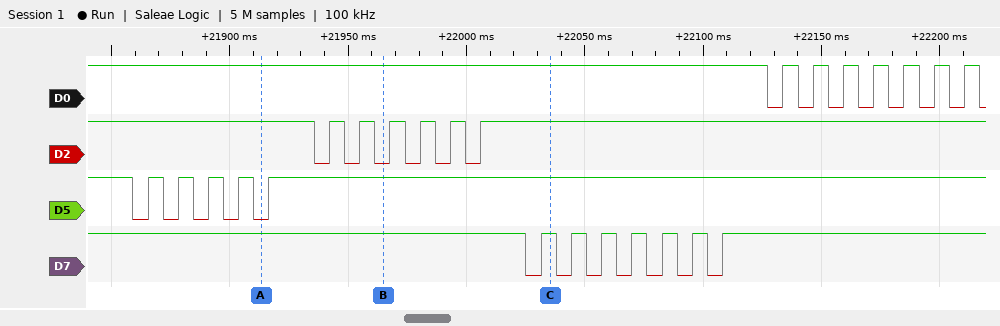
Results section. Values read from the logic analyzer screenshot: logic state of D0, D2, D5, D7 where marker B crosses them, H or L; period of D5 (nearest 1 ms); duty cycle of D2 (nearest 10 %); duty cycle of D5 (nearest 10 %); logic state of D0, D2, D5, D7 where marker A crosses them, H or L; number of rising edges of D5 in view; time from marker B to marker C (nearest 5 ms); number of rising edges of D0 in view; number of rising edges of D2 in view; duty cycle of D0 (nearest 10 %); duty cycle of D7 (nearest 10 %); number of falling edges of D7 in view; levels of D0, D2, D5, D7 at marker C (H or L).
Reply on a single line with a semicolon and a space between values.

D0=H, D2=L, D5=H, D7=H; 13 ms; 50 %; 50 %; D0=H, D2=H, D5=L, D7=H; 5; 70 ms; 7; 6; 50 %; 50 %; 7; D0=H, D2=H, D5=H, D7=H
